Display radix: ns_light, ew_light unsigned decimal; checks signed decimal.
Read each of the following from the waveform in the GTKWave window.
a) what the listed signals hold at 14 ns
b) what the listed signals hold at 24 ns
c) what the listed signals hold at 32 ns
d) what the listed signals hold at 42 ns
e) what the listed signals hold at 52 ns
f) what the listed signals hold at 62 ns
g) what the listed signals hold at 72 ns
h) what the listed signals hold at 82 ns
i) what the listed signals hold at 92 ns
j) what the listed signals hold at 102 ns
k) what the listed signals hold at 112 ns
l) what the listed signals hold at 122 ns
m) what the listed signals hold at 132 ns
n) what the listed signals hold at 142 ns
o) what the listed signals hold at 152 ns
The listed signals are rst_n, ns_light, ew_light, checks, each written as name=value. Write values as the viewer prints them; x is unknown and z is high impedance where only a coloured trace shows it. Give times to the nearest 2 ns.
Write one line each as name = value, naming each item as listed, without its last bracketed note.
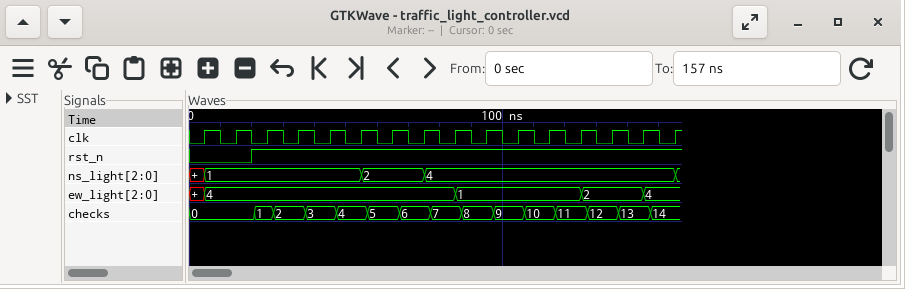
what the listed signals hold at 14 ns = rst_n=0, ns_light=1, ew_light=4, checks=0
what the listed signals hold at 24 ns = rst_n=1, ns_light=1, ew_light=4, checks=1
what the listed signals hold at 32 ns = rst_n=1, ns_light=1, ew_light=4, checks=2
what the listed signals hold at 42 ns = rst_n=1, ns_light=1, ew_light=4, checks=3
what the listed signals hold at 52 ns = rst_n=1, ns_light=1, ew_light=4, checks=4
what the listed signals hold at 62 ns = rst_n=1, ns_light=2, ew_light=4, checks=5
what the listed signals hold at 72 ns = rst_n=1, ns_light=2, ew_light=4, checks=6
what the listed signals hold at 82 ns = rst_n=1, ns_light=4, ew_light=4, checks=7
what the listed signals hold at 92 ns = rst_n=1, ns_light=4, ew_light=1, checks=8
what the listed signals hold at 102 ns = rst_n=1, ns_light=4, ew_light=1, checks=9
what the listed signals hold at 112 ns = rst_n=1, ns_light=4, ew_light=1, checks=10
what the listed signals hold at 122 ns = rst_n=1, ns_light=4, ew_light=1, checks=11
what the listed signals hold at 132 ns = rst_n=1, ns_light=4, ew_light=2, checks=12
what the listed signals hold at 142 ns = rst_n=1, ns_light=4, ew_light=2, checks=13
what the listed signals hold at 152 ns = rst_n=1, ns_light=4, ew_light=4, checks=14
